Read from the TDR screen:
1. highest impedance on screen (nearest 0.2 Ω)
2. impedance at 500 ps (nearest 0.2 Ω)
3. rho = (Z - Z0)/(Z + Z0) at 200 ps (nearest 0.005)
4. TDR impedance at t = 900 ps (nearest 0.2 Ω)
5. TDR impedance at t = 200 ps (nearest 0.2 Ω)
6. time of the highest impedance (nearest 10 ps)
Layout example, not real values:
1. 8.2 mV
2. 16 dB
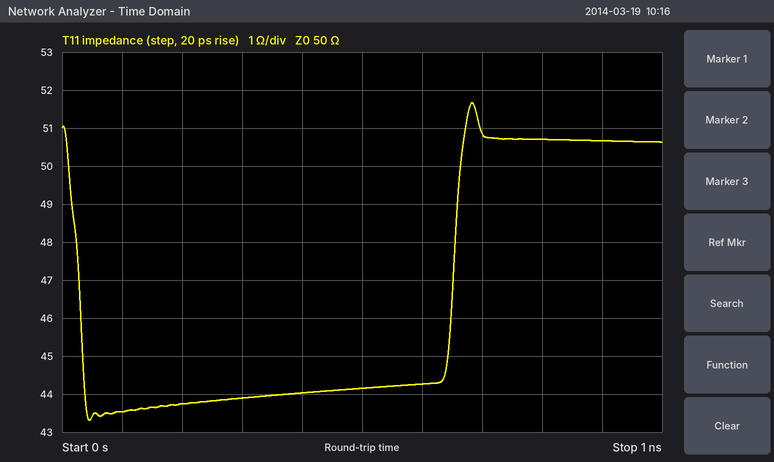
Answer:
1. 51.6 Ω
2. 44.2 Ω
3. -0.065
4. 50.6 Ω
5. 43.8 Ω
6. 680 ps
